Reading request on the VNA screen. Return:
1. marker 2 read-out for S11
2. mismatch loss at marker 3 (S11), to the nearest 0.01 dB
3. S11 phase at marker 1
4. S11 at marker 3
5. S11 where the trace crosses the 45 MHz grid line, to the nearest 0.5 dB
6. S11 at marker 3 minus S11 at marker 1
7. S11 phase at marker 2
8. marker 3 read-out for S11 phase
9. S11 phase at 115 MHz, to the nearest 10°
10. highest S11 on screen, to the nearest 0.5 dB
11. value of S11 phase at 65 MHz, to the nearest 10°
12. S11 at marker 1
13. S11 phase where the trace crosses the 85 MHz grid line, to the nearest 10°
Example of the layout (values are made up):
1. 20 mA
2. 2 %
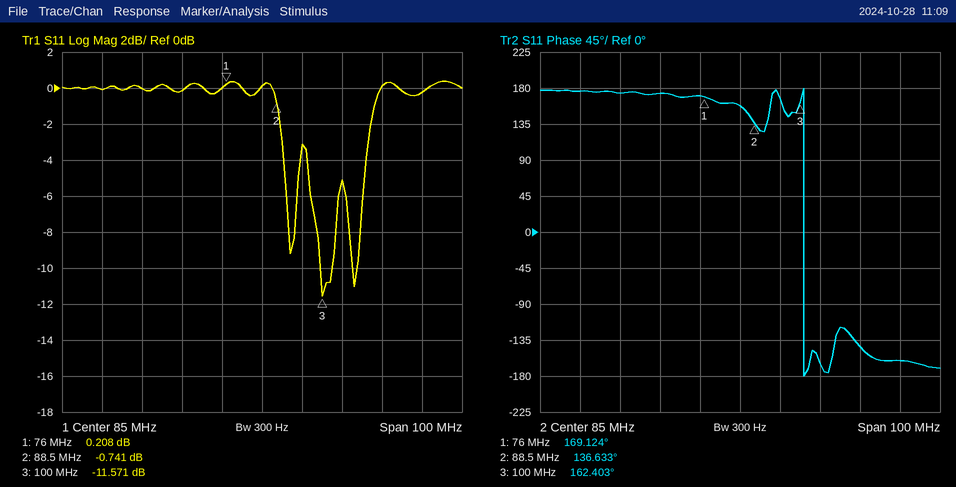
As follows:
1. -0.741 dB
2. 0.31 dB
3. 169.124°
4. -11.571 dB
5. 0.0 dB
6. -11.779 dB
7. 136.633°
8. 162.403°
9. -140°
10. 0.5 dB
11. 170°
12. 0.208 dB
13. 160°
